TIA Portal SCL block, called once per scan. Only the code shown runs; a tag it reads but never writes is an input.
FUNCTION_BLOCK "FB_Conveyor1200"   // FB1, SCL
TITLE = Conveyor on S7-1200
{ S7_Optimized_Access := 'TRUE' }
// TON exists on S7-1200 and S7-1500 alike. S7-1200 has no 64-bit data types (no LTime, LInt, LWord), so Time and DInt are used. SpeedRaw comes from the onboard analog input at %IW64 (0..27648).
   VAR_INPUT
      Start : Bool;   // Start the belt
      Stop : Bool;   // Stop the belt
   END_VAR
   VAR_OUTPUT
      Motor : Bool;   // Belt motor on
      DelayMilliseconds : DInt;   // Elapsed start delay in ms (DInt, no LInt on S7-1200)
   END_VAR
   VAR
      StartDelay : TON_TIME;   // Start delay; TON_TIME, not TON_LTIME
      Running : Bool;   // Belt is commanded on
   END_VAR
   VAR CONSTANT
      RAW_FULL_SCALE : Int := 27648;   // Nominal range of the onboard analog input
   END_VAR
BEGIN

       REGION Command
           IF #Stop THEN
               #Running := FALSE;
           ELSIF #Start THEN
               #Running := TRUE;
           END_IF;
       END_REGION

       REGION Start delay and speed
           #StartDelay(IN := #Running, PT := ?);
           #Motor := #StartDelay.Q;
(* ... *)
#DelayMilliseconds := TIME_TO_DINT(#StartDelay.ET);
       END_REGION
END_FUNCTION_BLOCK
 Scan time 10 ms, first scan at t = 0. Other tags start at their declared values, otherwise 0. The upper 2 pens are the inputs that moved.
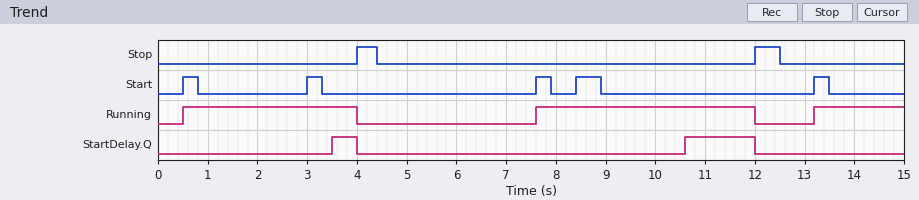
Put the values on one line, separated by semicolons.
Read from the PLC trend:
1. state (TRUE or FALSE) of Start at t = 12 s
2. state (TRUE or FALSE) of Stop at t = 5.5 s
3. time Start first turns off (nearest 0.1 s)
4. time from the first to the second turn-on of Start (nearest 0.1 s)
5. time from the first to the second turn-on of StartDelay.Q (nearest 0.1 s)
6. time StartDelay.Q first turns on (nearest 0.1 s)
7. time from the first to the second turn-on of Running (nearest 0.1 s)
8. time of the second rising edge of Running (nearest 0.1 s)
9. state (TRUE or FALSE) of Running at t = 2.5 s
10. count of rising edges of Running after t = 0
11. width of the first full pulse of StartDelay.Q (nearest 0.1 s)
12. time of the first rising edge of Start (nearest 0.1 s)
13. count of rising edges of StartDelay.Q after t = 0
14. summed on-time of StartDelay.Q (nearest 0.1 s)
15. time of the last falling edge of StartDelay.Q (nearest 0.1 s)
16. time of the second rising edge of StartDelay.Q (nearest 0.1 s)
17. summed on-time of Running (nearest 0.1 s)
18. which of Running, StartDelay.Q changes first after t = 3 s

FALSE; FALSE; 0.8 s; 2.5 s; 7.1 s; 3.5 s; 7.1 s; 7.6 s; TRUE; 3; 0.5 s; 0.5 s; 2; 1.9 s; 12.0 s; 10.6 s; 9.7 s; StartDelay.Q
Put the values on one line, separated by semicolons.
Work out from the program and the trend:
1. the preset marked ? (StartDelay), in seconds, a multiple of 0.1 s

3.0 s
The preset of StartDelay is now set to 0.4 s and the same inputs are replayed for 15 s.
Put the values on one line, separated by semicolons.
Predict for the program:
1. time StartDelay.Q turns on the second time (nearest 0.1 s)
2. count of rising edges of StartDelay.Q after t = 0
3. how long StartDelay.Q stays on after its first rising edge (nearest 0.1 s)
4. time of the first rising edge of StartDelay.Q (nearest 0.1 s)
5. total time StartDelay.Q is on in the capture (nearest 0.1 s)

8.0 s; 3; 3.1 s; 0.9 s; 8.5 s
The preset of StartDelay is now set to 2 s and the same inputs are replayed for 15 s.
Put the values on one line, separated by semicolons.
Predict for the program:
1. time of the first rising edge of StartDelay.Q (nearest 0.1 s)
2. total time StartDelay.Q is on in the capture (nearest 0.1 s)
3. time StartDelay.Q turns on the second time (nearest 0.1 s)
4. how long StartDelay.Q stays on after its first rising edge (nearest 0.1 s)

2.5 s; 3.9 s; 9.6 s; 1.5 s
